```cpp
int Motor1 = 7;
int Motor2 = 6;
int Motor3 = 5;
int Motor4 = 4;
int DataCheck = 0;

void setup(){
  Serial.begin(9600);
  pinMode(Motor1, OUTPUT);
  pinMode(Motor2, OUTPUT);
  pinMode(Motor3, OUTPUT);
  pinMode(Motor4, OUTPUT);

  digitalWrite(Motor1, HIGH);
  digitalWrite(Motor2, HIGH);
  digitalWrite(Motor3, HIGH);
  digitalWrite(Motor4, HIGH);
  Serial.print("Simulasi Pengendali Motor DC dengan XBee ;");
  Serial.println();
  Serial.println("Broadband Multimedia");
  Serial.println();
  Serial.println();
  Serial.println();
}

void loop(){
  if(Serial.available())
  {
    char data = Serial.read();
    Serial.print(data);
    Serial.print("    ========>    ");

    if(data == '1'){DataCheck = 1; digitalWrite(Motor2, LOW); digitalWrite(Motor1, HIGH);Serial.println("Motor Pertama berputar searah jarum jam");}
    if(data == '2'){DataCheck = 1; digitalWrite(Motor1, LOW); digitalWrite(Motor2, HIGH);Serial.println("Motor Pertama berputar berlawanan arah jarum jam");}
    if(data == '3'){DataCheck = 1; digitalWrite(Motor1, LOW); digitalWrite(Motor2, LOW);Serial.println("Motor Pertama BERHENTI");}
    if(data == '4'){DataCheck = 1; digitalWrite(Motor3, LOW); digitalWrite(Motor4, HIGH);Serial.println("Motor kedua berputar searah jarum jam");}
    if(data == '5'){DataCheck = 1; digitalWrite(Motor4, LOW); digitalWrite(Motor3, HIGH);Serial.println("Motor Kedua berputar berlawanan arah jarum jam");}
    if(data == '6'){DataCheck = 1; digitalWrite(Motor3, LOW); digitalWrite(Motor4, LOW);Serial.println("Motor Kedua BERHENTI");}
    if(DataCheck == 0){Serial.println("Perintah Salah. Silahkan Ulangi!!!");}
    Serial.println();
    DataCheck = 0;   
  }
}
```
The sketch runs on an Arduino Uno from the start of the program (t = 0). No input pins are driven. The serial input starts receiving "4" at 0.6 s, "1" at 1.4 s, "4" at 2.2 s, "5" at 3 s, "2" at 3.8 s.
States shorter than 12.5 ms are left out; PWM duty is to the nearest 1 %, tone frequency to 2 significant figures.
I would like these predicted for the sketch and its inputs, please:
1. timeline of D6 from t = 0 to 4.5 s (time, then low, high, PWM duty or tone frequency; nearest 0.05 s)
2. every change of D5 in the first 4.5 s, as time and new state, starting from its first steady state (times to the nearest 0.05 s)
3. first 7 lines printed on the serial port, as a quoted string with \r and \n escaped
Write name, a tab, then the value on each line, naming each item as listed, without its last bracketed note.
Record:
timeline of D6 from t = 0 to 4.5 s	0 s high; 1.4 s low; 3.8 s high
every change of D5 in the first 4.5 s, as time and new state, starting from its first steady state	0 s high; 0.6 s low; 3 s high
first 7 lines printed on the serial port, as a quoted string with \r and \n escaped	"Simulasi Pengendali Motor DC dengan XBee ;\r\nBroadband Multimedia\r\n\r\n\r\n\r\n4    ========>    Motor kedua berputar searah jarum jam\r\n\r\n"
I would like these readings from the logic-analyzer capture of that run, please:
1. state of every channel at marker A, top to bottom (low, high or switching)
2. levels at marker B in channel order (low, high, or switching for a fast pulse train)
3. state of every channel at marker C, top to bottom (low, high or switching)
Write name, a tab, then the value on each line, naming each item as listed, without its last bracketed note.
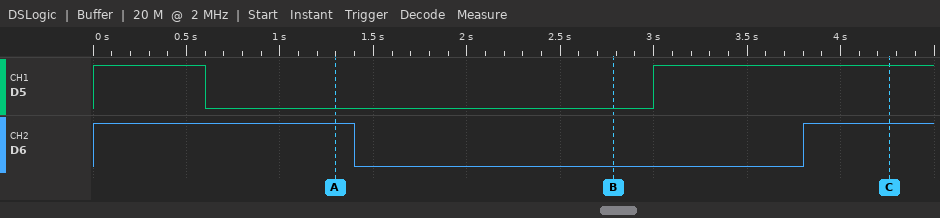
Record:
state of every channel at marker A, top to bottom	D5 low, D6 high
levels at marker B in channel order	D5 low, D6 low
state of every channel at marker C, top to bottom	D5 high, D6 high
